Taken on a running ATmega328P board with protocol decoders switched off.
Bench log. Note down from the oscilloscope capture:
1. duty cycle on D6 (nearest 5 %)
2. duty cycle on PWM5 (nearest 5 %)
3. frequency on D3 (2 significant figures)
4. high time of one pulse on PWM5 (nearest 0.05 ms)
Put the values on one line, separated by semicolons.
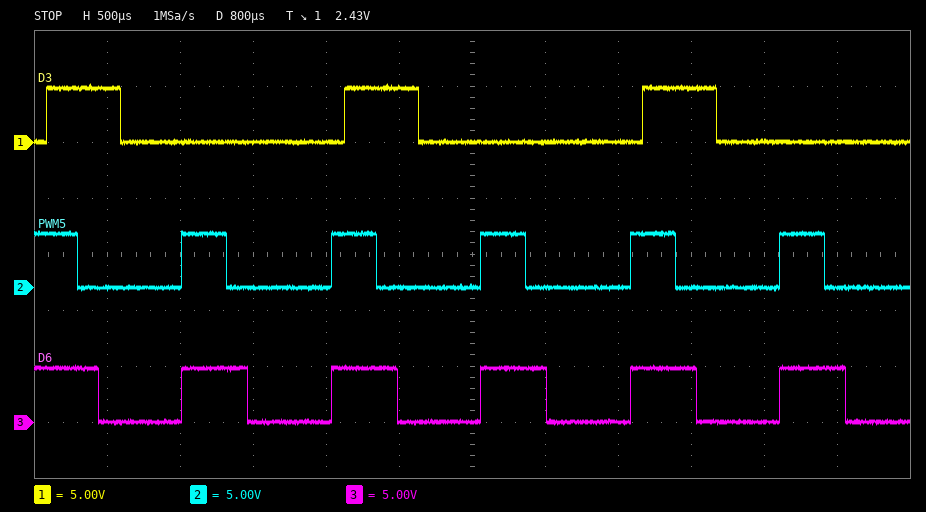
45 %; 30 %; 490 Hz; 0.30 ms
